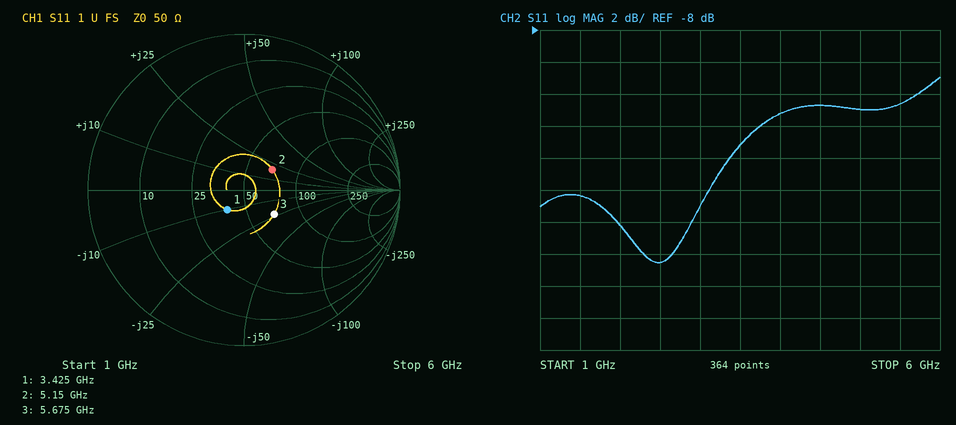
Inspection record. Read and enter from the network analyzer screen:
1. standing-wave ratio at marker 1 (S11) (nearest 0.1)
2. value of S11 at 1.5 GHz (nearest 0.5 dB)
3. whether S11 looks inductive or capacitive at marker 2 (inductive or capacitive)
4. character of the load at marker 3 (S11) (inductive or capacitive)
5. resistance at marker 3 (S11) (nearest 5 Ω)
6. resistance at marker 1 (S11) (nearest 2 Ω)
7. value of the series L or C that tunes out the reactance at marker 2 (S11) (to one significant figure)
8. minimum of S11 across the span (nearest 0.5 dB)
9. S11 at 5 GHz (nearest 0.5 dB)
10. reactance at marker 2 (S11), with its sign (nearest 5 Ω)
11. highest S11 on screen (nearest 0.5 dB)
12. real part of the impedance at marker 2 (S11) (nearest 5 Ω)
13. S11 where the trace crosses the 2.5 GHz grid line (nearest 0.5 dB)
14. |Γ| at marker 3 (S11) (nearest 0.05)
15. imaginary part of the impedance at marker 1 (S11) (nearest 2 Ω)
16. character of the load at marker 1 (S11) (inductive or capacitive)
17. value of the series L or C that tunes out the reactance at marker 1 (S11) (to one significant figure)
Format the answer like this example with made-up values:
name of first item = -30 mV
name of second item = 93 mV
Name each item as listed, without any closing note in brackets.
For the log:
standing-wave ratio at marker 1 (S11) = 1.4
value of S11 at 1.5 GHz = -18.5 dB
whether S11 looks inductive or capacitive at marker 2 = inductive
character of the load at marker 3 (S11) = capacitive
resistance at marker 3 (S11) = 70 Ω
resistance at marker 1 (S11) = 40 Ω
value of the series L or C that tunes out the reactance at marker 2 (S11) = 2 pF
minimum of S11 across the span = -22.5 dB
S11 at 5 GHz = -13.0 dB
reactance at marker 2 (S11), with its sign = +20 Ω
highest S11 on screen = -11.0 dB
real part of the impedance at marker 2 (S11) = 70 Ω
S11 where the trace crosses the 2.5 GHz grid line = -22.5 dB
|Γ| at marker 3 (S11) = 0.25
imaginary part of the impedance at marker 1 (S11) = -10 Ω
character of the load at marker 1 (S11) = capacitive
value of the series L or C that tunes out the reactance at marker 1 (S11) = 500 pH
